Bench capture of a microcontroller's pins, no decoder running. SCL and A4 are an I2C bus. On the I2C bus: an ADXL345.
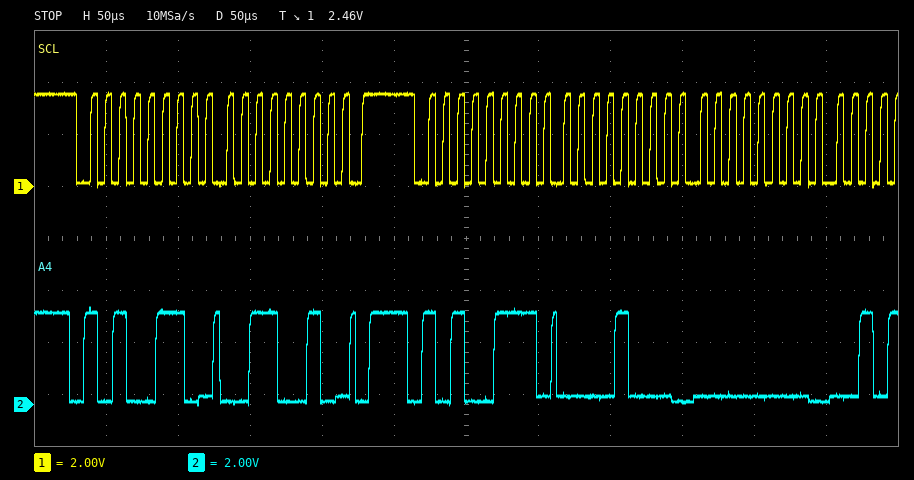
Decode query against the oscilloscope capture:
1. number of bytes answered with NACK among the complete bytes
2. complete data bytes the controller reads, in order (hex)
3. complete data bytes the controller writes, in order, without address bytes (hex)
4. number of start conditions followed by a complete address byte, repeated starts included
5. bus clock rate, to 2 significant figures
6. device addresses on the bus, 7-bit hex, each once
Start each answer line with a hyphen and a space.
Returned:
- 0
- 08 00
- 32
- 2
- 100 kHz
- 0x53
